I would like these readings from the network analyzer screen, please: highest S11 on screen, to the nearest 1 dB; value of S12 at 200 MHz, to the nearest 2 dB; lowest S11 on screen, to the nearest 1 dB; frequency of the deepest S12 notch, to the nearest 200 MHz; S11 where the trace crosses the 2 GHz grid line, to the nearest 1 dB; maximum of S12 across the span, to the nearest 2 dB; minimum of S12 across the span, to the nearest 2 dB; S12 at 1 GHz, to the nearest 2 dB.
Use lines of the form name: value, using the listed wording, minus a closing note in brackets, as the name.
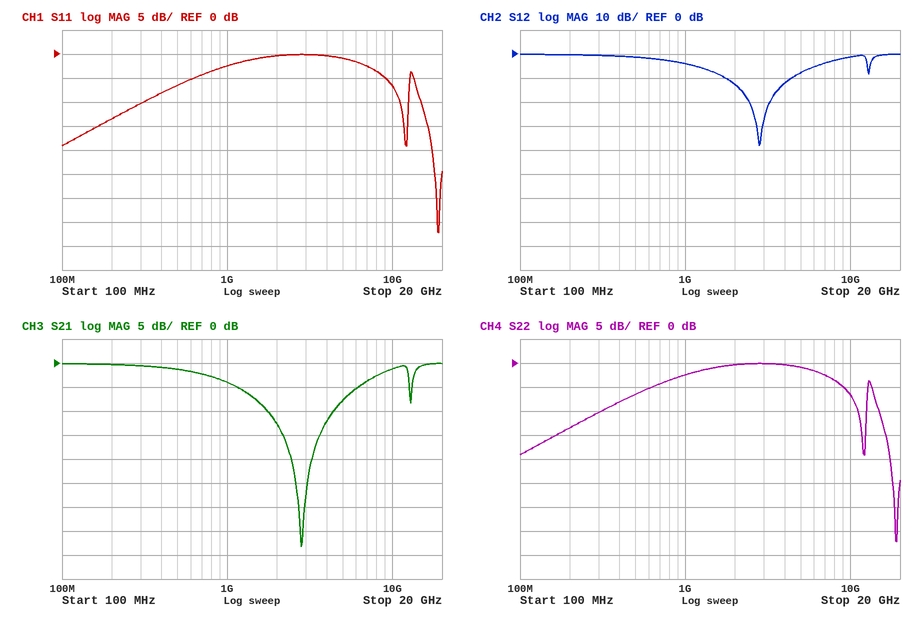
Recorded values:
highest S11 on screen, to the nearest 1 dB: 0 dB
value of S12 at 200 MHz, to the nearest 2 dB: 0 dB
lowest S11 on screen, to the nearest 1 dB: -37 dB
frequency of the deepest S12 notch, to the nearest 200 MHz: 2.8 GHz
S11 where the trace crosses the 2 GHz grid line, to the nearest 1 dB: 0 dB
maximum of S12 across the span, to the nearest 2 dB: 0 dB
minimum of S12 across the span, to the nearest 2 dB: -38 dB
S12 at 1 GHz, to the nearest 2 dB: -4 dB
